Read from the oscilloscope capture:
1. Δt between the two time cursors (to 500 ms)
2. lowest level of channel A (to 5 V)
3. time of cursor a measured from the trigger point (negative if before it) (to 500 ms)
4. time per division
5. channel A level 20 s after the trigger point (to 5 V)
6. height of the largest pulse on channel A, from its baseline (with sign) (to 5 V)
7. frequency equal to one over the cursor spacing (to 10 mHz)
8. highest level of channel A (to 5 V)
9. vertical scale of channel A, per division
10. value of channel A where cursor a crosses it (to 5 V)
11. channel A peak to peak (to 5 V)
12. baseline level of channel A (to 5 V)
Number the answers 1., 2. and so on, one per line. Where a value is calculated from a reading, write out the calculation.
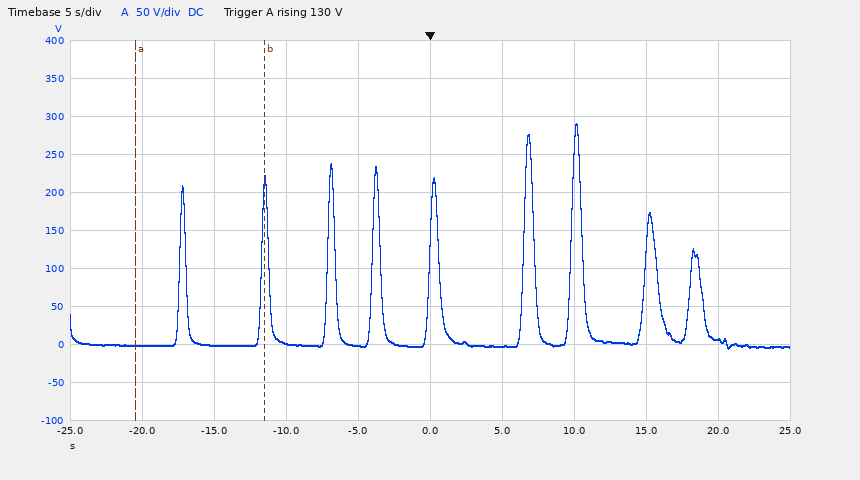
1. 9.0 s
2. -5 V
3. -20.5 s
4. 5 s
5. 5 V
6. 290 V − (0 V) = +290 V
7. 1 / 9.0 s ≈ 110 mHz
8. 290 V
9. 50 V
10. 0 V
11. 290 V − (-5 V) = 295 V
12. 0 V
